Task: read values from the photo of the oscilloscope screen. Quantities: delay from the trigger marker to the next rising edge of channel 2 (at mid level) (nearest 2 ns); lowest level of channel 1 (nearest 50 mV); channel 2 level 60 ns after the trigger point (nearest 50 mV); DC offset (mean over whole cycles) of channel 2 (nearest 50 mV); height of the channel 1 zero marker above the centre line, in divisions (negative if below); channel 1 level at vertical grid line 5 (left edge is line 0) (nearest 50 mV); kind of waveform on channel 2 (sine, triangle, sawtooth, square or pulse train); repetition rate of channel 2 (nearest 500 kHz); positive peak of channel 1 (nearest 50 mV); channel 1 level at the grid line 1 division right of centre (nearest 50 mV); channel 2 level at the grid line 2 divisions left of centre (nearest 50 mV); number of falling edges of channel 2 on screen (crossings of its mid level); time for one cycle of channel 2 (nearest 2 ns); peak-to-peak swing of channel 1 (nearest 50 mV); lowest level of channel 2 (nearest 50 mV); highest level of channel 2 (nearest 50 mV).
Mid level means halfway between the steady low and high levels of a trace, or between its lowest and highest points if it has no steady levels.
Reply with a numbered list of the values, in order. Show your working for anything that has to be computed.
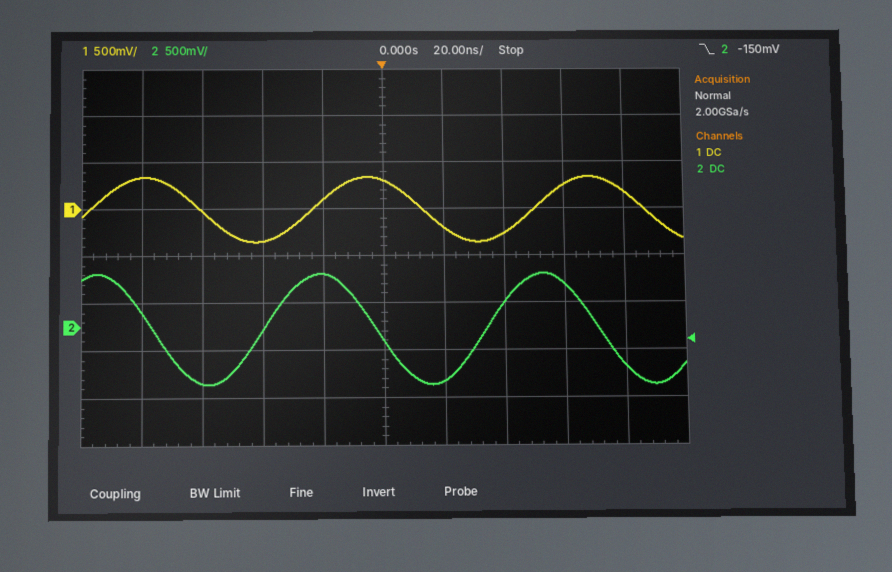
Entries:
1. 34 ns
2. -350 mV
3. 450 mV
4. (550 mV + (-600 mV)) / 2 ≈ 0 mV
5. +1.0 div
6. 300 mV
7. sine
8. 1 / 74 ns ≈ 13.5 MHz
9. 350 mV
10. -200 mV
11. -50 mV
12. 3
13. 74 ns
14. 350 mV − (-350 mV) = 700 mV
15. -600 mV
16. 550 mV
